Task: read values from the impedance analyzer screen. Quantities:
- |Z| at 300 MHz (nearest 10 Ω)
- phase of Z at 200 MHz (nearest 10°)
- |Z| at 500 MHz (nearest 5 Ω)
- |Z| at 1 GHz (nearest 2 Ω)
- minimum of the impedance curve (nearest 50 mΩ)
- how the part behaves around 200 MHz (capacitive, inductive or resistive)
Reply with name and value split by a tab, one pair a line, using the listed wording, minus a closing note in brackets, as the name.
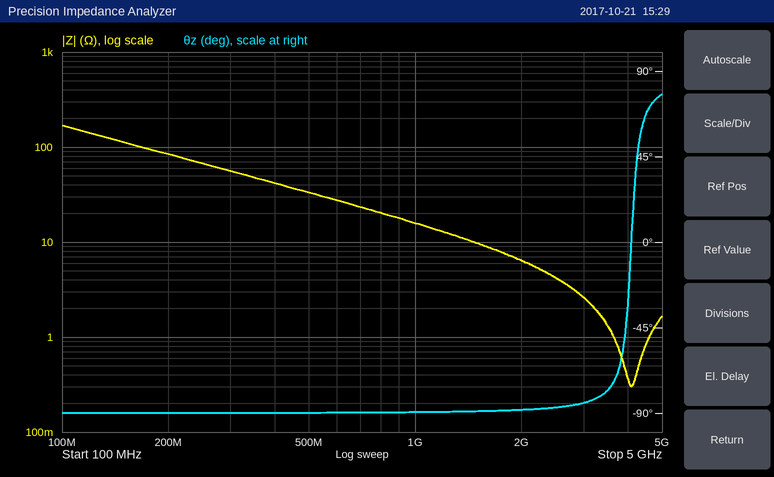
|Z| at 300 MHz	60 Ω
phase of Z at 200 MHz	-90°
|Z| at 500 MHz	35 Ω
|Z| at 1 GHz	16 Ω
minimum of the impedance curve	300 mΩ
how the part behaves around 200 MHz	capacitive
